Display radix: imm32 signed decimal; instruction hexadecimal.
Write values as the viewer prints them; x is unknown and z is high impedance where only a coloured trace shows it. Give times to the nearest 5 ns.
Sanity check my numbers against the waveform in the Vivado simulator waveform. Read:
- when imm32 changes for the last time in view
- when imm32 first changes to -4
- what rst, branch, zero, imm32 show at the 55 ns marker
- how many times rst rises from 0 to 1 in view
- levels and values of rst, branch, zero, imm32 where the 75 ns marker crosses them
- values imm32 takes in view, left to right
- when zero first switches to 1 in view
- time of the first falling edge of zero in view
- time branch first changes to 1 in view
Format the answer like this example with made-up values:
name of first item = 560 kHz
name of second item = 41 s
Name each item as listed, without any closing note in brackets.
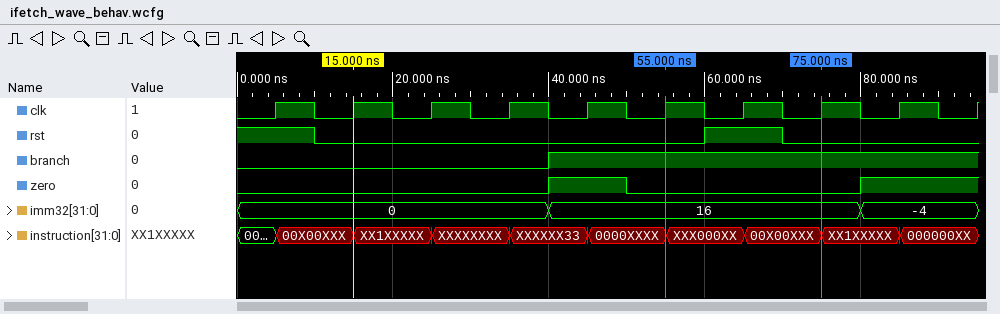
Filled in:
when imm32 changes for the last time in view = 80 ns
when imm32 first changes to -4 = 80 ns
what rst, branch, zero, imm32 show at the 55 ns marker = rst=0, branch=1, zero=0, imm32=16
how many times rst rises from 0 to 1 in view = 1
levels and values of rst, branch, zero, imm32 where the 75 ns marker crosses them = rst=0, branch=1, zero=0, imm32=16
values imm32 takes in view, left to right = 0, 16, -4
when zero first switches to 1 in view = 40 ns
time of the first falling edge of zero in view = 50 ns
time branch first changes to 1 in view = 40 ns
